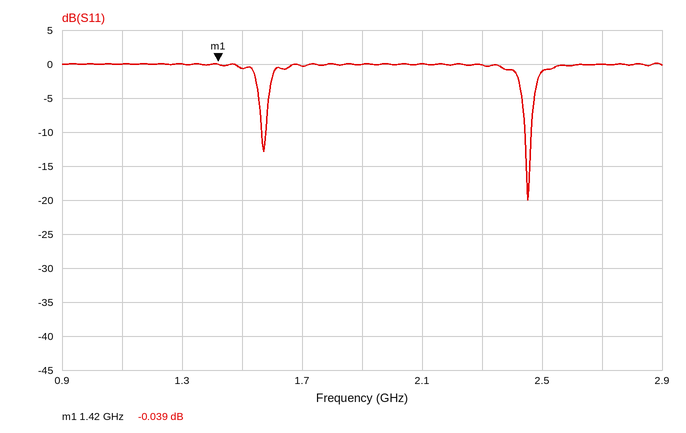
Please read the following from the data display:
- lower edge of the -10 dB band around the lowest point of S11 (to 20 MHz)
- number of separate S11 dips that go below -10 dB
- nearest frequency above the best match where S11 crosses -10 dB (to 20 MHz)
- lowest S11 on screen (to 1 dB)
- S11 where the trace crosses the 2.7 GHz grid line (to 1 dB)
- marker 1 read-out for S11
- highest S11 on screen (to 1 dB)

2.44 GHz
2
2.46 GHz
-20 dB
0 dB
-0.039 dB
0 dB
